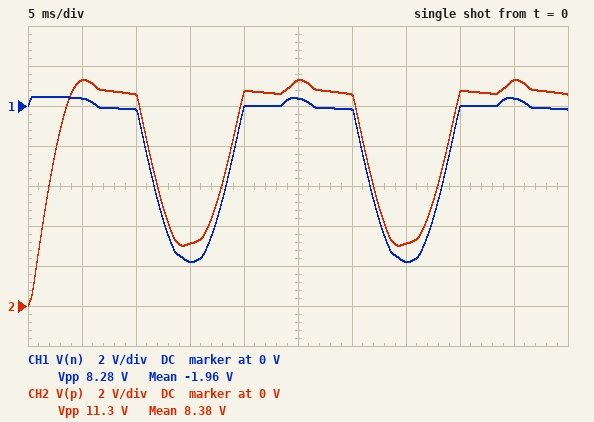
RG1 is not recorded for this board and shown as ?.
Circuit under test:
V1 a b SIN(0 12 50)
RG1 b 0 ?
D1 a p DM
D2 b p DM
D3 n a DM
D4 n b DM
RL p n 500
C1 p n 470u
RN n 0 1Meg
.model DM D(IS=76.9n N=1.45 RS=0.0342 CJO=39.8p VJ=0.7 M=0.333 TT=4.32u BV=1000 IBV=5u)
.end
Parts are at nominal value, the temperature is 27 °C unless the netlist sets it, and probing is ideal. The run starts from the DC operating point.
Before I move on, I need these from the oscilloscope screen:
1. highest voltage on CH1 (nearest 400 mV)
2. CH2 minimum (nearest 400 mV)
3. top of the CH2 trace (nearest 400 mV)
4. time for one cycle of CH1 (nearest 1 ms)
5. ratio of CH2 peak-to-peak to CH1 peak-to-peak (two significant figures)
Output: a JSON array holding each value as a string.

["400 mV", "0 V", "11.2 V", "20 ms", "1.4"]
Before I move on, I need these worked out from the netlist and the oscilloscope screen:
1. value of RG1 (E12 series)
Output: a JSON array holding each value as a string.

["470 kΩ"]
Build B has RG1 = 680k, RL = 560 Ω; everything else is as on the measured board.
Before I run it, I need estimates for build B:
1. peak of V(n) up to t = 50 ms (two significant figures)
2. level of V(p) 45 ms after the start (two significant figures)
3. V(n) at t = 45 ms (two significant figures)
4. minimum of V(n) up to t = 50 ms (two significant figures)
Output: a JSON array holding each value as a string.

["410 mV", "11 V", "320 mV", "-6.8 V"]
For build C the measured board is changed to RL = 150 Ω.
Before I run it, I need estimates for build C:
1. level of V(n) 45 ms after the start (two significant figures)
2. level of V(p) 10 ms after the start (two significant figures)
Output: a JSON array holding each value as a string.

["380 mV", "10 V"]
